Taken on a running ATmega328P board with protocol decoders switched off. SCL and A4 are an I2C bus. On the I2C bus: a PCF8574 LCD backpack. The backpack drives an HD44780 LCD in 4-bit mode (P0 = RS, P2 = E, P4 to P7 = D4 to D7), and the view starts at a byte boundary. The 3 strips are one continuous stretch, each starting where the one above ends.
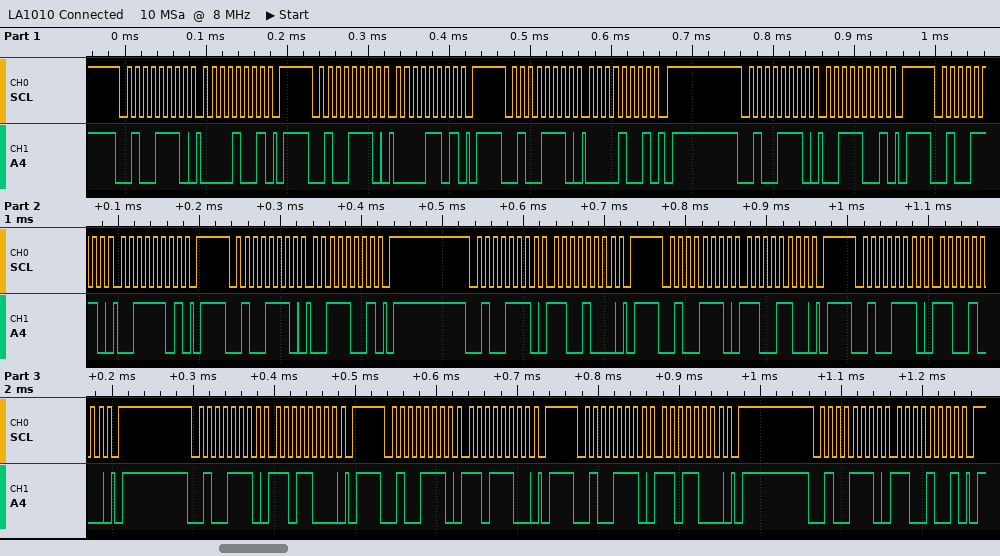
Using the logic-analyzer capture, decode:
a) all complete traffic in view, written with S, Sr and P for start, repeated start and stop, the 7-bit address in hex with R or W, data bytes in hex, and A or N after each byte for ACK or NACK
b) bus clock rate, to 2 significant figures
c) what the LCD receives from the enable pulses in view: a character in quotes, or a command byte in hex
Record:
S 27W A 09 A P S 27W A 0D A P S 27W A 09 A P S 27W A 39 A P S 27W A 3D A P S 27W A 39 A P S 27W A C8 A P S 27W A CC A P S 27W A C8 A P S 27W A D8 A P S 27W A DC A P S 27W A D8 A P S 27W A C9 A P
100 kHz
data 0x03 0xCD
